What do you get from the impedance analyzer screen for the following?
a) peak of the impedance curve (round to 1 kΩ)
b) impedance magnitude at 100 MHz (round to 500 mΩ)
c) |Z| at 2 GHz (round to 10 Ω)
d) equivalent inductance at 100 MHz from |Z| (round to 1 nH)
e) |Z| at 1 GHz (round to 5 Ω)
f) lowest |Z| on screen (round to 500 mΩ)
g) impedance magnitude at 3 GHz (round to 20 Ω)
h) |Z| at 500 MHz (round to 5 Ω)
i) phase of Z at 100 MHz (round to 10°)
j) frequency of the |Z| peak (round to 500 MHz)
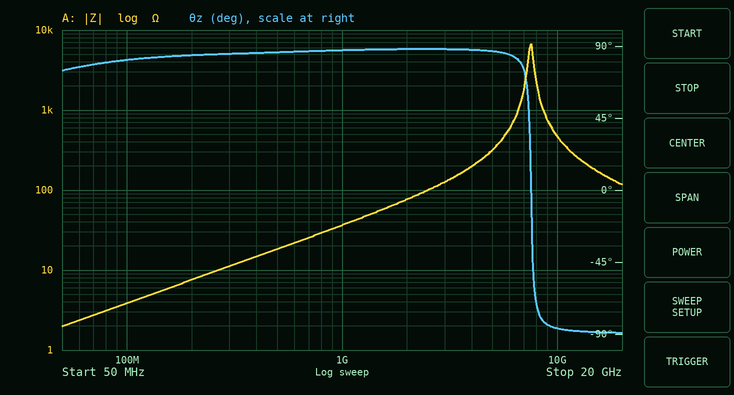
7 kΩ
4.0 Ω
80 Ω
6 nH
35 Ω
2.0 Ω
120 Ω
20 Ω
80°
7.5 GHz
